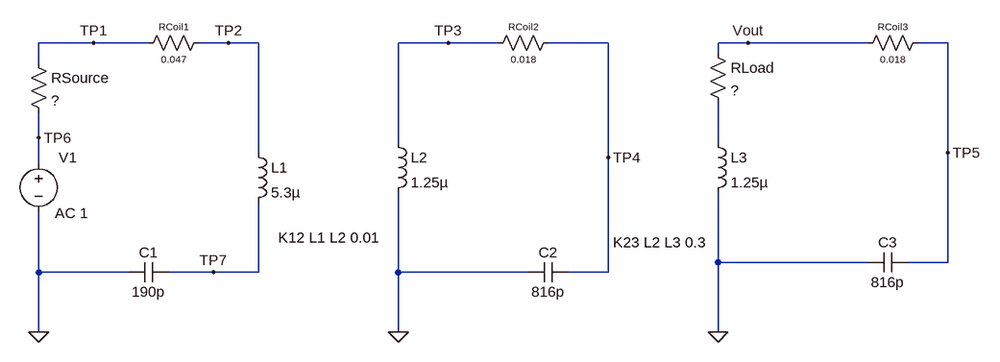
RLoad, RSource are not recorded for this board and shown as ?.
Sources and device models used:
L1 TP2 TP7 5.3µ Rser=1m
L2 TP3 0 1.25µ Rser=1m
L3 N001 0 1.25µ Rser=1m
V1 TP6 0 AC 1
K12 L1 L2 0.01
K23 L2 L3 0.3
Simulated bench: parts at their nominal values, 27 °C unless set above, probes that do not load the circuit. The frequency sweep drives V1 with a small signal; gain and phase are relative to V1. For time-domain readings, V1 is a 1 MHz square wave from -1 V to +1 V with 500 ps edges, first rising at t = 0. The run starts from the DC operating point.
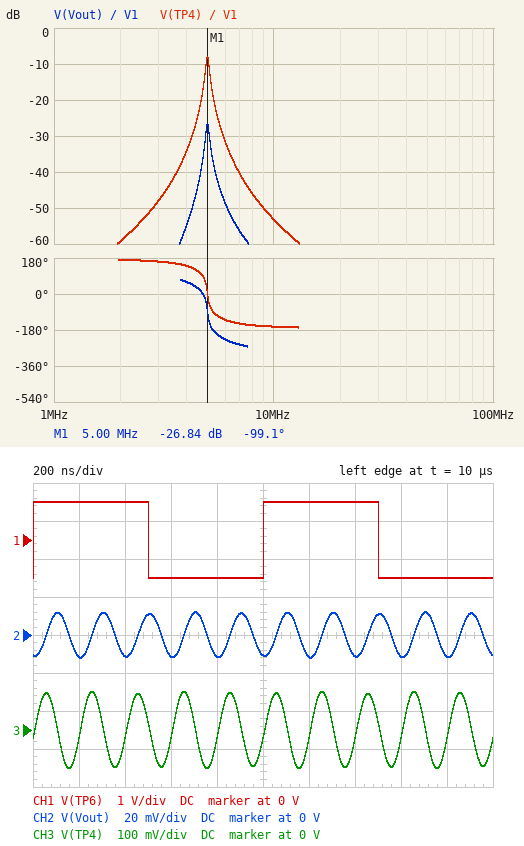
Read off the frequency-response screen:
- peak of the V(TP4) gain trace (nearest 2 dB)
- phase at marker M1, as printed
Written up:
-8 dB
-99.1 deg
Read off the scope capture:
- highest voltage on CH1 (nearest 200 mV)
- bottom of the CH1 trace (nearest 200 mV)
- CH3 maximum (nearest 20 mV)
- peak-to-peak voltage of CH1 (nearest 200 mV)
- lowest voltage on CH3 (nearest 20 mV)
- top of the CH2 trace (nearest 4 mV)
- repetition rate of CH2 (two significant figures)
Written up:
1.0 V
-1.0 V
100 mV
2.0 V
-100 mV
12 mV
5.0 MHz
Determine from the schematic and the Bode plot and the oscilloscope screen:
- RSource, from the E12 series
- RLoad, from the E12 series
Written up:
56 Ω
100 Ω
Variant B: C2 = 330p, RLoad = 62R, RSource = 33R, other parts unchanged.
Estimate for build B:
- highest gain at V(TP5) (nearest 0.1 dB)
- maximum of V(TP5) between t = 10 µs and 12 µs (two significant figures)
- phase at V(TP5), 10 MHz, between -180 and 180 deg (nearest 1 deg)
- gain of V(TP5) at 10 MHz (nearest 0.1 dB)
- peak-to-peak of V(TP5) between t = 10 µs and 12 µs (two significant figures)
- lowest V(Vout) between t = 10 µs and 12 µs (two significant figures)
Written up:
-38.5 dB
1.9 mV
64 deg
-57.6 dB
3.8 mV
-1.9 mV
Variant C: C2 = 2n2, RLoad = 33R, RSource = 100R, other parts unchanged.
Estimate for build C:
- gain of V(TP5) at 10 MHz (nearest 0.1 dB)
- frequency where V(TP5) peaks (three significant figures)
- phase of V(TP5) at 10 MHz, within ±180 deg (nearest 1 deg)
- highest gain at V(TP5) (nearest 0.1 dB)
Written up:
-63.9 dB
2.99 MHz
55 deg
-29.4 dB
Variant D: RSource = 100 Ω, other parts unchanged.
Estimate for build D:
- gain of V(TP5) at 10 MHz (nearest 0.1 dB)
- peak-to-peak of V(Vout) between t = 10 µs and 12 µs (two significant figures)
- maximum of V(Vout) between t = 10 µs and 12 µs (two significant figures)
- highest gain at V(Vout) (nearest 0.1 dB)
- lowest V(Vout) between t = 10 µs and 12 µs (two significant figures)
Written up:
-67.5 dB
14 mV
6.8 mV
-31.6 dB
-6.8 mV
